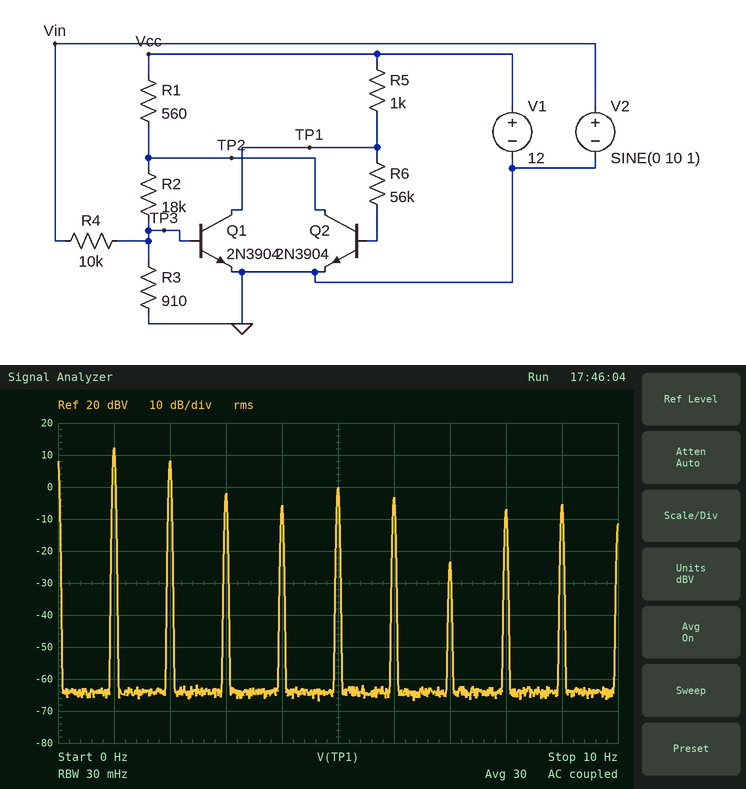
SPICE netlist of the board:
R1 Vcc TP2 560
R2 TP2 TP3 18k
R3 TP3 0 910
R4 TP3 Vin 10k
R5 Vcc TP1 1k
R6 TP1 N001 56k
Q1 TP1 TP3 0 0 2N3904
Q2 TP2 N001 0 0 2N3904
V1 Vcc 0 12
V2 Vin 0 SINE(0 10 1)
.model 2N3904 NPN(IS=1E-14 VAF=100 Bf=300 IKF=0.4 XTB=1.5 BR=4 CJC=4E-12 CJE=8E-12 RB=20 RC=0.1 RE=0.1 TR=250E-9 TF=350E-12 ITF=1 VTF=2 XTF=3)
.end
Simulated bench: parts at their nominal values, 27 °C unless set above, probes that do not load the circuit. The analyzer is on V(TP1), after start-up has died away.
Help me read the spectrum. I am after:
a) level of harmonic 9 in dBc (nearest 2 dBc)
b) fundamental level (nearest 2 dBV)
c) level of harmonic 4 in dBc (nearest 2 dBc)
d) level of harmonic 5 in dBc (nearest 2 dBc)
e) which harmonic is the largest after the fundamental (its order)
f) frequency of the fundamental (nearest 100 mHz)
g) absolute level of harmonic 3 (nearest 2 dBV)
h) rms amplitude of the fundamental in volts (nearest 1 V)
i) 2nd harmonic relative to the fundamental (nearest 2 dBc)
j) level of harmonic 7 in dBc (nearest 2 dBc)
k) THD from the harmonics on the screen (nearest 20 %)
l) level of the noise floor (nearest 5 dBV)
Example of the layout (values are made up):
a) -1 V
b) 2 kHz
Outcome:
a) -18 dBc
b) 12 dBV
c) -18 dBc
d) -12 dBc
e) 2
f) 1.0 Hz
g) -2 dBV
h) 4 V
i) -4 dBc
j) -36 dBc
k) 80 %
l) -65 dBV
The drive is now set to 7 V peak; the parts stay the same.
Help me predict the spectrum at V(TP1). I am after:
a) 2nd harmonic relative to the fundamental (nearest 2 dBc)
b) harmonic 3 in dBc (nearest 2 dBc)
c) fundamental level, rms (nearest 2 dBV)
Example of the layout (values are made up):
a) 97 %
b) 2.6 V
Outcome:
a) 0 dBc
b) -2 dBc
c) -48 dBV
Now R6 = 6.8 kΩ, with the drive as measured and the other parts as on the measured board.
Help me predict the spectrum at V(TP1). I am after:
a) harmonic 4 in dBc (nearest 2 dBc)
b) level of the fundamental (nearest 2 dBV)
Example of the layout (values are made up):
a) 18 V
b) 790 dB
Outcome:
a) -20 dBc
b) 12 dBV
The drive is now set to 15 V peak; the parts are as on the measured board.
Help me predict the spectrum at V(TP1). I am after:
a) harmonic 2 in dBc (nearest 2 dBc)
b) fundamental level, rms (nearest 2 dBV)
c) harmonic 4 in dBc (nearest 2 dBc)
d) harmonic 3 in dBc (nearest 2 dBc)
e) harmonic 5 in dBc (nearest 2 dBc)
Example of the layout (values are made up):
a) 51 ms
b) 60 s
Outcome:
a) -8 dBc
b) 14 dBV
c) -12 dBc
d) -18 dBc
e) -20 dBc
